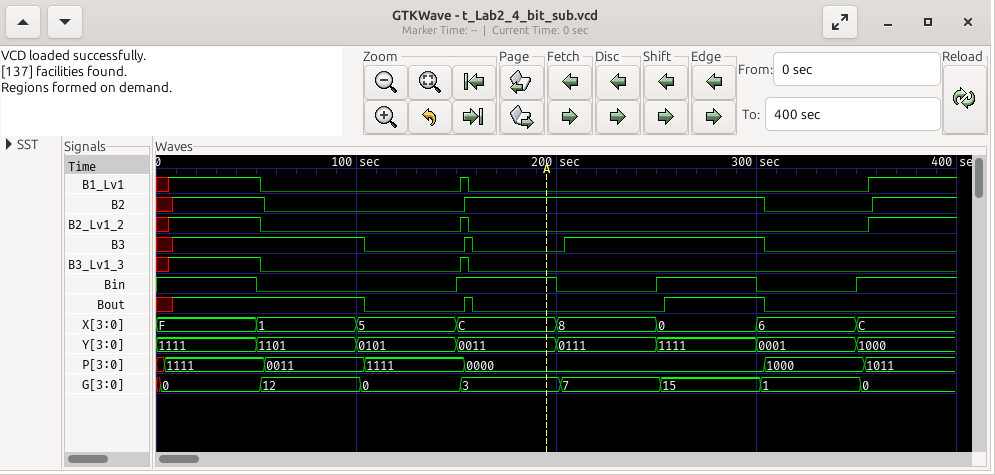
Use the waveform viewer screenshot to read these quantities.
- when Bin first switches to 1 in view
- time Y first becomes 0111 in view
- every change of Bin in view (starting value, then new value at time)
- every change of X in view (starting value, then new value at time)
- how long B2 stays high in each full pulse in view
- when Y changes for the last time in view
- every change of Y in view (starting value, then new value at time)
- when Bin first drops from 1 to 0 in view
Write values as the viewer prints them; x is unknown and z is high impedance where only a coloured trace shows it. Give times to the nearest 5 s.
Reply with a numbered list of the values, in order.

1. 150 s
2. 200 s
3. 1, 0 at 50 s, 1 at 150 s, 0 at 200 s, 1 at 250 s, 0 at 300 s, 1 at 350 s
4. F, 1 at 50 s, 5 at 100 s, C at 150 s, 8 at 200 s, 0 at 250 s, 6 at 300 s, C at 350 s
5. 150 s
6. 350 s
7. 1111, 1101 at 50 s, 0101 at 100 s, 0011 at 150 s, 0111 at 200 s, 1111 at 250 s, 0001 at 300 s, 1000 at 350 s
8. 50 s
